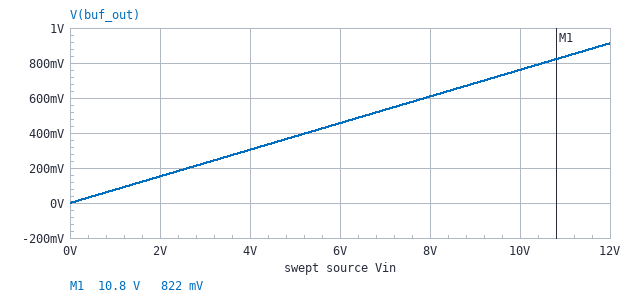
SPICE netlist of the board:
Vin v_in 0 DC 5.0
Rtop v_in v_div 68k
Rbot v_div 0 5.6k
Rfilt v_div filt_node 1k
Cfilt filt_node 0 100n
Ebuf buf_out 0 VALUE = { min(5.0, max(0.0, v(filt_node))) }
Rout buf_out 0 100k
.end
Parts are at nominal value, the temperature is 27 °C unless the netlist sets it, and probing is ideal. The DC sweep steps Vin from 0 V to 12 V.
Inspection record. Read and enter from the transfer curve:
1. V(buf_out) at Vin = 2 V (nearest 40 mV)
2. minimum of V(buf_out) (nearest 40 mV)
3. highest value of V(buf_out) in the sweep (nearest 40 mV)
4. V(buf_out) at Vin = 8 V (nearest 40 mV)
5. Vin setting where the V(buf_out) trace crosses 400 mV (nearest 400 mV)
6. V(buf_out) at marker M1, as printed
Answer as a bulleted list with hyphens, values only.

- 160 mV
- 0 V
- 920 mV
- 600 mV
- 5.2 V
- 822 mV
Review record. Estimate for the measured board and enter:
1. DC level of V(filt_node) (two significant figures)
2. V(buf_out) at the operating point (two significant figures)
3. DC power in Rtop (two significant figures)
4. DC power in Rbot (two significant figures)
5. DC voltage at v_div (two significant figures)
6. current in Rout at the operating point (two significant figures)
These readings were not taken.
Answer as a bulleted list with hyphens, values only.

- 380 mV
- 380 mV
- 310 µW
- 26 µW
- 380 mV
- 3.8 µA
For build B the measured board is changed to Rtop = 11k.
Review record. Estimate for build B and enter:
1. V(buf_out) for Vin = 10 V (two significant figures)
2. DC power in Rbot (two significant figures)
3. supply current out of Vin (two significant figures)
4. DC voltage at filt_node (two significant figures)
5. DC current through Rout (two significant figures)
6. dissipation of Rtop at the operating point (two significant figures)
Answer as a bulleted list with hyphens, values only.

- 3.4 V
- 510 µW
- 300 µA
- 1.7 V
- 17 µA
- 1.0 mW
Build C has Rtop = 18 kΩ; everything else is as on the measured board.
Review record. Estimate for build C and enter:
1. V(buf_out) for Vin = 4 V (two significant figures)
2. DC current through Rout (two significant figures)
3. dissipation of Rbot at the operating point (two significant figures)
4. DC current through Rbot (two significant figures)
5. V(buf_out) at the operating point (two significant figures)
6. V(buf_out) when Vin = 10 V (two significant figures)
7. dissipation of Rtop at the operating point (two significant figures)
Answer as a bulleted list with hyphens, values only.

- 950 mV
- 12 µA
- 250 µW
- 210 µA
- 1.2 V
- 2.4 V
- 810 µW
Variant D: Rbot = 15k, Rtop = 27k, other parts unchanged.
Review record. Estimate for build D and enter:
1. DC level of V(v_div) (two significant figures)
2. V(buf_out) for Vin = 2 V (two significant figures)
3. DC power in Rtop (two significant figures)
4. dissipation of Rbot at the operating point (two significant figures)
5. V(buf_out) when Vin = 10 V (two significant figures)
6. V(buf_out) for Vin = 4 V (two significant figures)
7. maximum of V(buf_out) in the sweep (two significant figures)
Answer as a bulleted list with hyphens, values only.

- 1.8 V
- 710 mV
- 380 µW
- 210 µW
- 3.6 V
- 1.4 V
- 4.3 V
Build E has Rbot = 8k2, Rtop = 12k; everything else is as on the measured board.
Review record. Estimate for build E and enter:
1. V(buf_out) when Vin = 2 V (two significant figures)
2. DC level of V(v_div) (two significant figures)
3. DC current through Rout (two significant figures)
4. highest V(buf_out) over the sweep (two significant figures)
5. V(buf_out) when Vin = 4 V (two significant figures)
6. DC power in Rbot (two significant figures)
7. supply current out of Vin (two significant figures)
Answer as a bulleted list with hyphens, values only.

- 810 mV
- 2.0 V
- 20 µA
- 4.9 V
- 1.6 V
- 500 µW
- 250 µA
